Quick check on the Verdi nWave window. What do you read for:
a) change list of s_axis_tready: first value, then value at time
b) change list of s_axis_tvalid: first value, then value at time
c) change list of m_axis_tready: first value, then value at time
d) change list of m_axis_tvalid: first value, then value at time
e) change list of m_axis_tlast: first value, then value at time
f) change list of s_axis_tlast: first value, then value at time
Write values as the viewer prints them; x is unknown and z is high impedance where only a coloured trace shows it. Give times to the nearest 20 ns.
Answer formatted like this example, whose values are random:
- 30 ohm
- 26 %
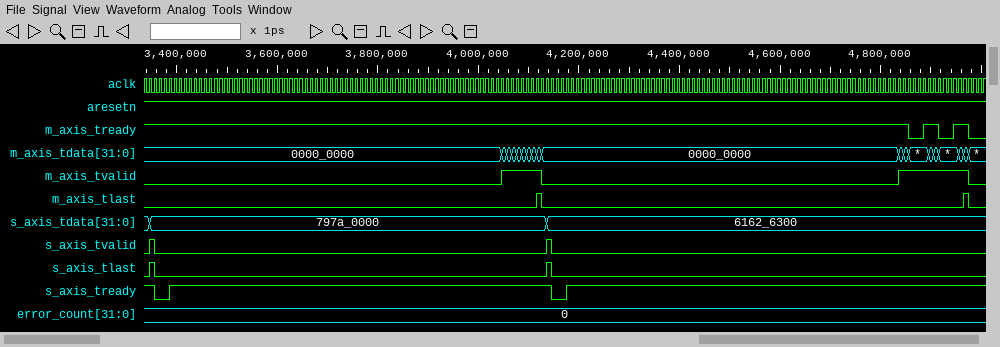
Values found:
- 1, 0 at 3360 ns, 1 at 3380 ns, 0 at 4140 ns, 1 at 4180 ns
- 0, 1 at 3340 ns, 0 at 3360 ns, 1 at 4140 ns, 0 at 4140 ns
- 1, 0 at 4860 ns, 1 at 4880 ns, 0 at 4920 ns, 1 at 4940 ns, 0 at 4980 ns
- 0, 1 at 4040 ns, 0 at 4120 ns, 1 at 4840 ns, 0 at 4980 ns
- 0, 1 at 4120 ns, 0 at 4120 ns, 1 at 4960 ns, 0 at 4980 ns
- 0, 1 at 3340 ns, 0 at 3360 ns, 1 at 4140 ns, 0 at 4140 ns
